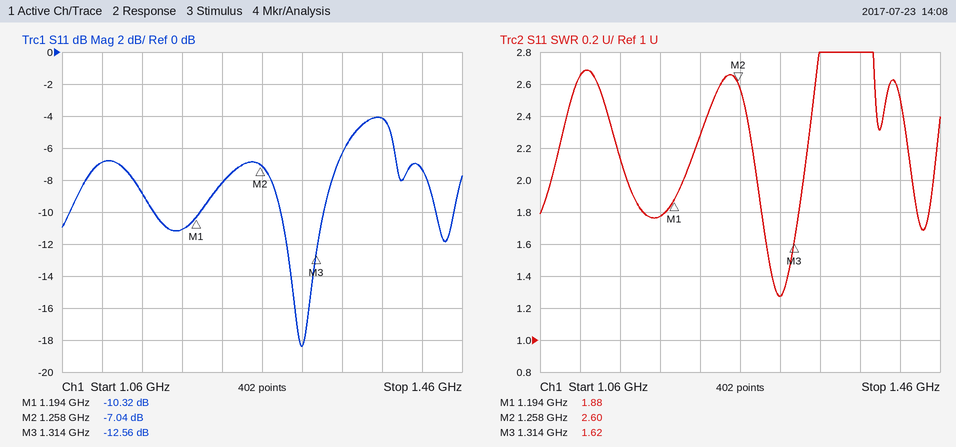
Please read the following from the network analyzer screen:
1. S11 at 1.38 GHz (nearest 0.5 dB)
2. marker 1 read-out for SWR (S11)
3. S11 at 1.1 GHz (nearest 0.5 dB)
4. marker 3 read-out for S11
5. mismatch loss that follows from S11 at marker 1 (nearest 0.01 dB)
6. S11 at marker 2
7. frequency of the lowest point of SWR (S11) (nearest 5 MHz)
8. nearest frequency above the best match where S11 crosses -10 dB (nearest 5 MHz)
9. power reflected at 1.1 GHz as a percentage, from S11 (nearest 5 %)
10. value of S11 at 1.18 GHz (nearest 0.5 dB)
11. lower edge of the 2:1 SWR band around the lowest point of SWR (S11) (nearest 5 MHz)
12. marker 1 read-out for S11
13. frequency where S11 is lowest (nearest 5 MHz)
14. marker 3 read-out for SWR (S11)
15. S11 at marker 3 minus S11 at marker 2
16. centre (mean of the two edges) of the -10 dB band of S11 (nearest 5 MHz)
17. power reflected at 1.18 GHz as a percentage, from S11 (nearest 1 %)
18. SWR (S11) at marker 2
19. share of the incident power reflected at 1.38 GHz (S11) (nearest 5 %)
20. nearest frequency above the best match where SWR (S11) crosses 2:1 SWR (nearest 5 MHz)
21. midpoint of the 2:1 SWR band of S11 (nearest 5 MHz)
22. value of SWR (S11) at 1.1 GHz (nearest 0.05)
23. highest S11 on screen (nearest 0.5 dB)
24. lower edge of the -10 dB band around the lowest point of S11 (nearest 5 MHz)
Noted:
-4.0 dB
1.88
-7.0 dB
-12.56 dB
0.42 dB
-7.04 dB
1.300 GHz
1.320 GHz
20 %
-11.0 dB
1.275 GHz
-10.32 dB
1.300 GHz
1.62
-5.52 dB
1.300 GHz
8 %
2.60
40 %
1.325 GHz
1.300 GHz
2.65
-4.0 dB
1.280 GHz
